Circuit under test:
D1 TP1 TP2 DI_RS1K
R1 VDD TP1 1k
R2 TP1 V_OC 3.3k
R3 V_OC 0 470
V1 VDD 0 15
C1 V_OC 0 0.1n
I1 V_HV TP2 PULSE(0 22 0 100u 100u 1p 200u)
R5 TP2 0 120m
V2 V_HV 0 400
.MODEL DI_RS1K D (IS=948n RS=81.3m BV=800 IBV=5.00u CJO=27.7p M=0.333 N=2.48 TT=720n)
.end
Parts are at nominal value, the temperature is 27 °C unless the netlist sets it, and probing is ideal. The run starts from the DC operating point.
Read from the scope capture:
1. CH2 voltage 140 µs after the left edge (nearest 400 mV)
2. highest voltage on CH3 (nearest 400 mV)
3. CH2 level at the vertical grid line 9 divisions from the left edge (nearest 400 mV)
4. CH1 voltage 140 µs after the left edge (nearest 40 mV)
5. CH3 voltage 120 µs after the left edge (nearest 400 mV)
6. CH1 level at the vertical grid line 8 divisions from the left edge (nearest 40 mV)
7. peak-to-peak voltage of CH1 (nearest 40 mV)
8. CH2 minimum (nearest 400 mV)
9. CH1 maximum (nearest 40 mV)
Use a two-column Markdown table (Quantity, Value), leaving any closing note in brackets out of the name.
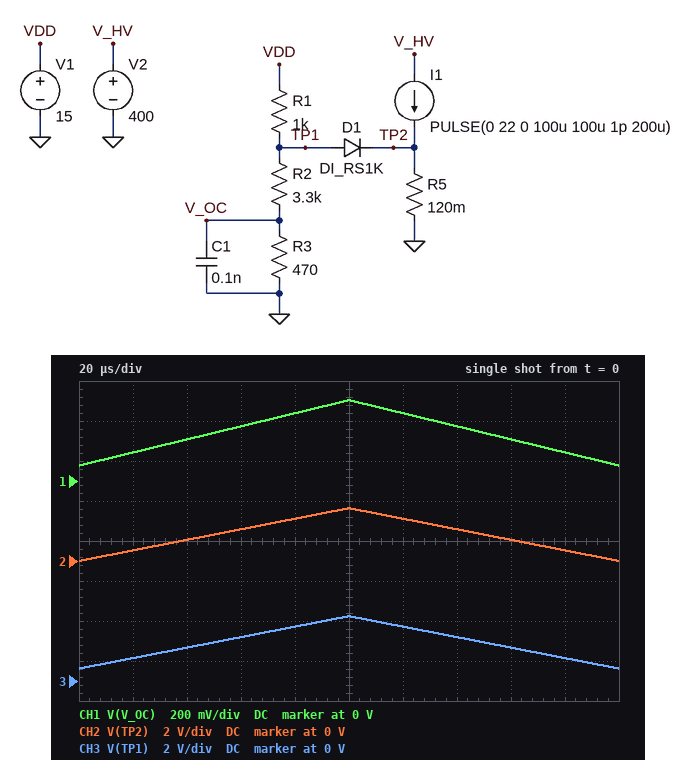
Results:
| Quantity | Value |
|---|---|
| CH2 voltage 140 µs after the left edge | 1.6 V |
| highest voltage on CH3 | 3.2 V |
| CH2 level at the vertical grid line 9 divisions from the left edge | 400 mV |
| CH1 voltage 140 µs after the left edge | 280 mV |
| CH3 voltage 120 µs after the left edge | 2.8 V |
| CH1 level at the vertical grid line 8 divisions from the left edge | 200 mV |
| peak-to-peak voltage of CH1 | 320 mV |
| CH2 minimum | 0 V |
| CH1 maximum | 400 mV |
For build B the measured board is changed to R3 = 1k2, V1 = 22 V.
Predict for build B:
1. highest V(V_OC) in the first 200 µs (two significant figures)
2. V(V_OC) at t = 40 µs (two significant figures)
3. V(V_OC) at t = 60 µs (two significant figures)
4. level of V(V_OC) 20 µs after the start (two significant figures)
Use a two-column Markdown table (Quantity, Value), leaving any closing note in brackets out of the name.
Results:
| Quantity | Value |
|---|---|
| highest V(V_OC) in the first 200 µs | 870 mV |
| V(V_OC) at t = 40 µs | 450 mV |
| V(V_OC) at t = 60 µs | 590 mV |
| level of V(V_OC) 20 µs after the start | 310 mV |
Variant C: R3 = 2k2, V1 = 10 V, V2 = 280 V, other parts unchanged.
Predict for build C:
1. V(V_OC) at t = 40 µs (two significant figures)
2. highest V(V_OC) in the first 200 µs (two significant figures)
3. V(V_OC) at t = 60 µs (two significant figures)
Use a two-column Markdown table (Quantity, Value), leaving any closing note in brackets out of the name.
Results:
| Quantity | Value |
|---|---|
| V(V_OC) at t = 40 µs | 650 mV |
| highest V(V_OC) in the first 200 µs | 1.3 V |
| V(V_OC) at t = 60 µs | 860 mV |
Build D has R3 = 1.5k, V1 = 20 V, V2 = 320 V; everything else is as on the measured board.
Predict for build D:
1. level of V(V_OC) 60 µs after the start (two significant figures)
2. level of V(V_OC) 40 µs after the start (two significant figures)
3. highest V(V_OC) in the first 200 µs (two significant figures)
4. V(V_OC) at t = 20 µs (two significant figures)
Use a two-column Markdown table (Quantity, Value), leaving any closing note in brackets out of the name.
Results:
| Quantity | Value |
|---|---|
| level of V(V_OC) 60 µs after the start | 690 mV |
| level of V(V_OC) 40 µs after the start | 530 mV |
| highest V(V_OC) in the first 200 µs | 1.0 V |
| V(V_OC) at t = 20 µs | 360 mV |
